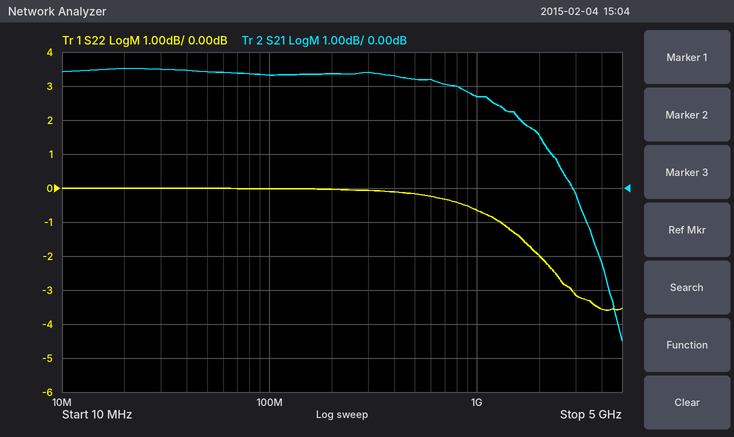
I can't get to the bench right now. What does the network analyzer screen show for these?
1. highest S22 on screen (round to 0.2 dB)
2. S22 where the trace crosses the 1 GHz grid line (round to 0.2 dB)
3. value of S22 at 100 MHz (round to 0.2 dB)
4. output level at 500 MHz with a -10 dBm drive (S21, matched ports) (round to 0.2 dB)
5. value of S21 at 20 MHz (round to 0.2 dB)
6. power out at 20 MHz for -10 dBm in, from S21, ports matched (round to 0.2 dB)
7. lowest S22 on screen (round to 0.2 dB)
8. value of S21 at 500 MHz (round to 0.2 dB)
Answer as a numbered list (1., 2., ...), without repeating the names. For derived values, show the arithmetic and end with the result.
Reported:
1. 0.0 dB
2. -0.6 dB
3. 0.0 dB
4. -10 dBm + (3.2 dB) = -6.8 dBm
5. 3.6 dB
6. -10 dBm + (3.6 dB) = -6.4 dBm
7. -3.6 dB
8. 3.2 dB
